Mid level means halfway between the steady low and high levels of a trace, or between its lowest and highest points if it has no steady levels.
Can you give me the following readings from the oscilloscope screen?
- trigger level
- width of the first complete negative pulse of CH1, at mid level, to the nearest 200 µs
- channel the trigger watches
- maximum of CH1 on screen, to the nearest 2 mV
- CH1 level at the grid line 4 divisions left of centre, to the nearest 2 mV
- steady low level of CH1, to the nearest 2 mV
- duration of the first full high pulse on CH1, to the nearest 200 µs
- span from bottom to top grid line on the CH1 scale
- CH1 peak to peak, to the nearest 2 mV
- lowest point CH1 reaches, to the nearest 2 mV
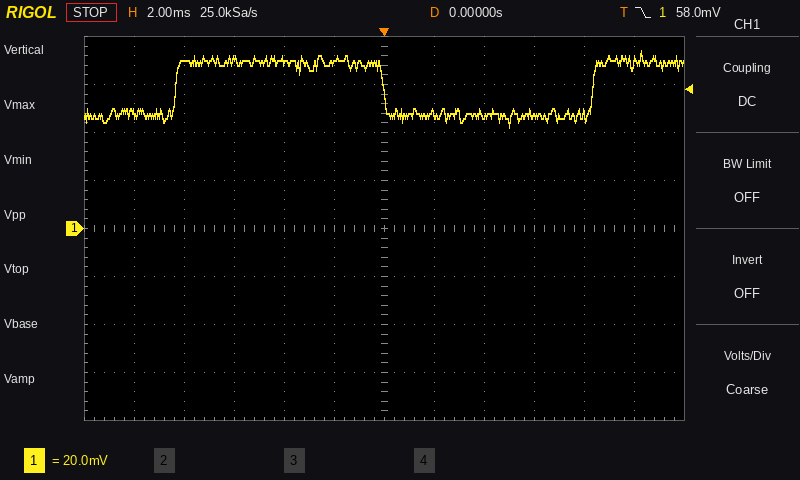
58.0 mV
8.4 ms
CH1
74 mV
70 mV
48 mV
8.4 ms
160 mV
32 mV
42 mV
